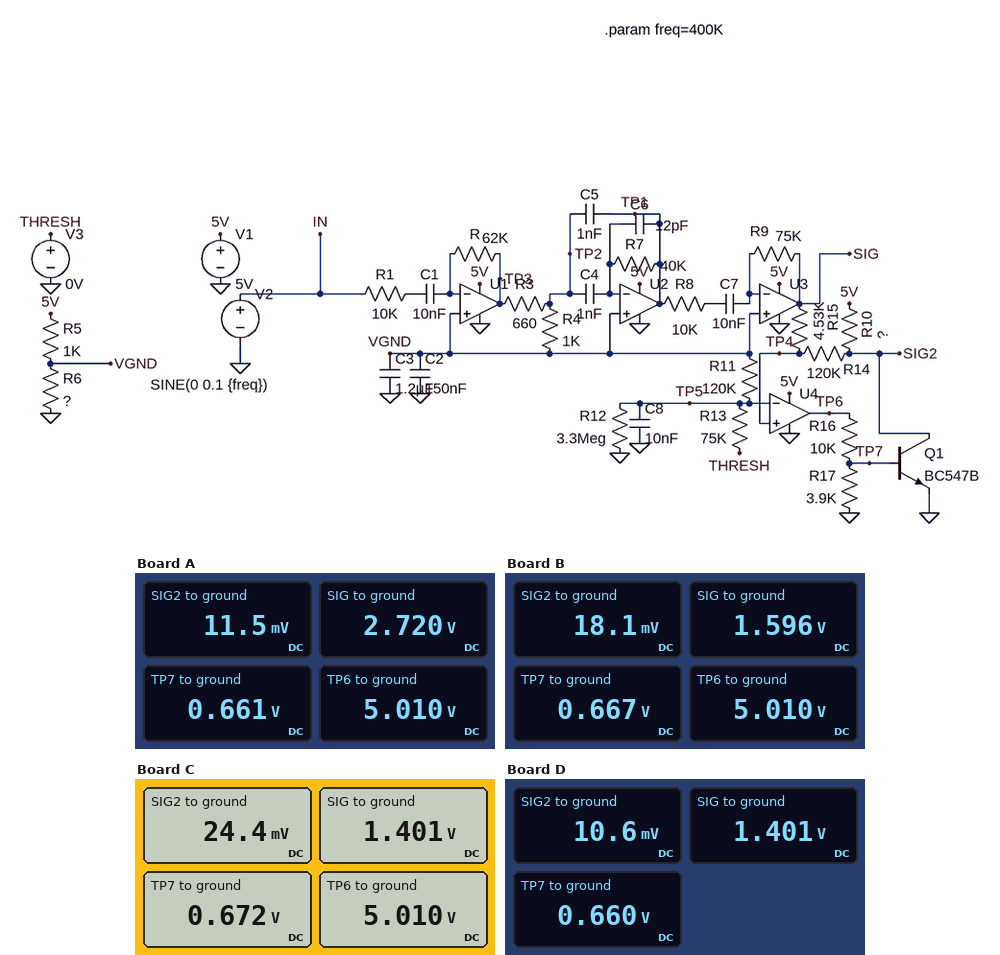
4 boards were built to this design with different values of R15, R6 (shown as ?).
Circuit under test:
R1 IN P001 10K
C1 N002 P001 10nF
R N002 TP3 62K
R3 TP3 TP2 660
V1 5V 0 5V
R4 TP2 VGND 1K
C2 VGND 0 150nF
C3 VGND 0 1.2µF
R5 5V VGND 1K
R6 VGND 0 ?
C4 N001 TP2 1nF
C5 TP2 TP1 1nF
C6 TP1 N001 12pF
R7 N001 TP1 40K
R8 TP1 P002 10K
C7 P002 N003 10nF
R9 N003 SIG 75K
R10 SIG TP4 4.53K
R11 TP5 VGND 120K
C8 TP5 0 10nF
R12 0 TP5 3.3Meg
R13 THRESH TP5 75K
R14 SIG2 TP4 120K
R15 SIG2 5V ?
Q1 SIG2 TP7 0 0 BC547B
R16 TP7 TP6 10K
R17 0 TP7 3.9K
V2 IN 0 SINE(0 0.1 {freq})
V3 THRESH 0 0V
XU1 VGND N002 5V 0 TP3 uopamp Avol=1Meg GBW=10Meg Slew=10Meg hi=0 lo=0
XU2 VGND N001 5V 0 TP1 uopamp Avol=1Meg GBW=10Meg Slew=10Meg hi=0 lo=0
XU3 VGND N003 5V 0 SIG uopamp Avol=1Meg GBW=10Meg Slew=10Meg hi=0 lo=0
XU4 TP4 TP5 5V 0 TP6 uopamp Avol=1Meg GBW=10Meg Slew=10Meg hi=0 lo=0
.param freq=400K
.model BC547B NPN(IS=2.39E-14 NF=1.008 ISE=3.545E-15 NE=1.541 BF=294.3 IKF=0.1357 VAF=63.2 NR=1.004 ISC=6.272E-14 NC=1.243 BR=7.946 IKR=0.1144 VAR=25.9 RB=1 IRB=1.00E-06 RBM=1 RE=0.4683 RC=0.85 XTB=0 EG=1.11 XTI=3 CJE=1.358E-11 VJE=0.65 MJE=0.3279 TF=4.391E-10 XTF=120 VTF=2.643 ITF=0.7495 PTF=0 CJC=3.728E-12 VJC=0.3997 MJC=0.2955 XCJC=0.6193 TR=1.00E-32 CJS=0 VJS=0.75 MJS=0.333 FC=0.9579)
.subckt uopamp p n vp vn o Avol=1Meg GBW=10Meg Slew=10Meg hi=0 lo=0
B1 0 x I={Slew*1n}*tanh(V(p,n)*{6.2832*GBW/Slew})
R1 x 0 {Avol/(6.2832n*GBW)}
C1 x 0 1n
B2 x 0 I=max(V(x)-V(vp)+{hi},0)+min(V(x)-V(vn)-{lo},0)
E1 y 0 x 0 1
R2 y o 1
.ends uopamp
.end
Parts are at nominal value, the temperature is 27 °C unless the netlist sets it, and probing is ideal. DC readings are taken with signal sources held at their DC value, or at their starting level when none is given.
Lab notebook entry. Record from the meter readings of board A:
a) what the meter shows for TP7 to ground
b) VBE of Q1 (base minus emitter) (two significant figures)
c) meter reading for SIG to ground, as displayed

0.661 V
660 mV
2.720 V
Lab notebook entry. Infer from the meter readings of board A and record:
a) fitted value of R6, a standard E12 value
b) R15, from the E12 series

1.2 kΩ
15 kΩ
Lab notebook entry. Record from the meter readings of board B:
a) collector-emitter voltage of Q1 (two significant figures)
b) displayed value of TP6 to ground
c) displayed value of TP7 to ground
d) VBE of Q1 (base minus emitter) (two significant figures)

18 mV
5.010 V
0.667 V
670 mV
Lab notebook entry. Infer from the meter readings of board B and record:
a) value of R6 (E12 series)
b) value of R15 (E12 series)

470 Ω
5.6 kΩ
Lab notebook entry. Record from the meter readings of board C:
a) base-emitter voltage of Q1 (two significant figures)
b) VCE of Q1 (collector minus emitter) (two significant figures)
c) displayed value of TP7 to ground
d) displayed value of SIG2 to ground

670 mV
24 mV
0.672 V
24.4 mV
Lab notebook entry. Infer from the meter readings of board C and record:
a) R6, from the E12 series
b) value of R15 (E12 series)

390 Ω
3.3 kΩ
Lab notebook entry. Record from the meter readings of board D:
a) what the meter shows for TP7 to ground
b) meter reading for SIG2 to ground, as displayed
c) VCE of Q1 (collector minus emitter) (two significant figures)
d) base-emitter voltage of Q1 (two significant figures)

0.660 V
10.6 mV
11 mV
660 mV
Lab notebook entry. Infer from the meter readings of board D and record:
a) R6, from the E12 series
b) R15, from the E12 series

390 Ω
18 kΩ
